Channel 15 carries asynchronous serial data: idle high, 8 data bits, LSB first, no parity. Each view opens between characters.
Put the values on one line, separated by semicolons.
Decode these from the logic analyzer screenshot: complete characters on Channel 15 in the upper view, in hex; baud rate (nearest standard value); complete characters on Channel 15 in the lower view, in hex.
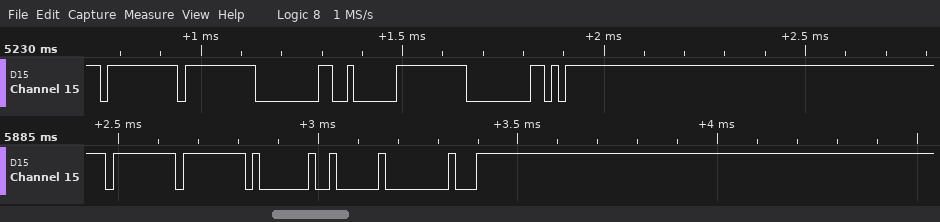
FF, FF, 00, 02, 00, FD; 57600 baud; FF, FF, 01, 02, 00, FC
